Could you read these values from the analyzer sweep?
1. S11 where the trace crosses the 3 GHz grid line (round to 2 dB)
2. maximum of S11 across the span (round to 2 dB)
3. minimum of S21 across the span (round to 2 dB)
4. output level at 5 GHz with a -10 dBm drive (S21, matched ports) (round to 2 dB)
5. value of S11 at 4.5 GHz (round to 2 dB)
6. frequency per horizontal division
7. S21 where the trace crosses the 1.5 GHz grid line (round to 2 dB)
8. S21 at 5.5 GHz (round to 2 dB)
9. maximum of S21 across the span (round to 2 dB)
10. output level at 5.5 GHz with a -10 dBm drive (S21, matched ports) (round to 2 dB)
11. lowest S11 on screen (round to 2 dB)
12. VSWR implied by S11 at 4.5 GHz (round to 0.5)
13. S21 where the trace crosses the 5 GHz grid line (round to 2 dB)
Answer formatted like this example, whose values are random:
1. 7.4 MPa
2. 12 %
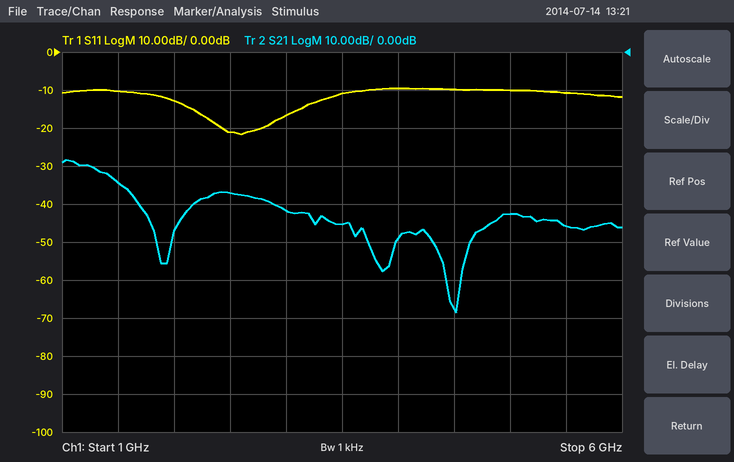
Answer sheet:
1. -16 dB
2. -10 dB
3. -68 dB
4. -52 dBm
5. -10 dB
6. 500 MHz
7. -34 dB
8. -46 dB
9. -28 dB
10. -56 dBm
11. -22 dB
12. 2.0
13. -42 dB
